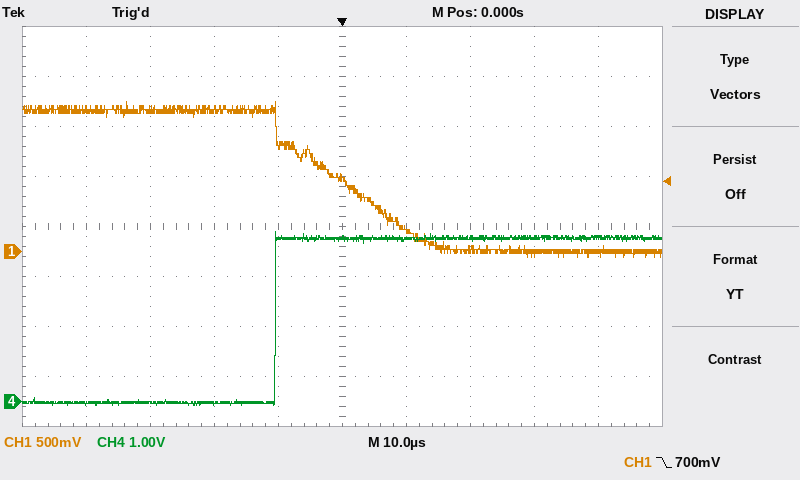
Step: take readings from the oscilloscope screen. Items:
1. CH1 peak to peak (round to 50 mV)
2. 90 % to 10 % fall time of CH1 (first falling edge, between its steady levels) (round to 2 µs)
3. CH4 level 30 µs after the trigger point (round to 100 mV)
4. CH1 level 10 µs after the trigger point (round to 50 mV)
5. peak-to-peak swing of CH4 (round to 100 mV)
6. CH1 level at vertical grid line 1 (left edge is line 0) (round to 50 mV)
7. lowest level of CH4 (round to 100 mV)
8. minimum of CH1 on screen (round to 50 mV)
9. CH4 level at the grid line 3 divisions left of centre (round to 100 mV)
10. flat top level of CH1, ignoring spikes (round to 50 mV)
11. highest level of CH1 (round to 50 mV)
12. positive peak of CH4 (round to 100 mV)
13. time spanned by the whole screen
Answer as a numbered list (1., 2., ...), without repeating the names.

1. 1.55 V
2. 22 µs
3. 3.3 V
4. 200 mV
5. 3.5 V
6. 1.40 V
7. -100 mV
8. -50 mV
9. 0.0 V
10. 1.40 V
11. 1.50 V
12. 3.4 V
13. 100 µs
